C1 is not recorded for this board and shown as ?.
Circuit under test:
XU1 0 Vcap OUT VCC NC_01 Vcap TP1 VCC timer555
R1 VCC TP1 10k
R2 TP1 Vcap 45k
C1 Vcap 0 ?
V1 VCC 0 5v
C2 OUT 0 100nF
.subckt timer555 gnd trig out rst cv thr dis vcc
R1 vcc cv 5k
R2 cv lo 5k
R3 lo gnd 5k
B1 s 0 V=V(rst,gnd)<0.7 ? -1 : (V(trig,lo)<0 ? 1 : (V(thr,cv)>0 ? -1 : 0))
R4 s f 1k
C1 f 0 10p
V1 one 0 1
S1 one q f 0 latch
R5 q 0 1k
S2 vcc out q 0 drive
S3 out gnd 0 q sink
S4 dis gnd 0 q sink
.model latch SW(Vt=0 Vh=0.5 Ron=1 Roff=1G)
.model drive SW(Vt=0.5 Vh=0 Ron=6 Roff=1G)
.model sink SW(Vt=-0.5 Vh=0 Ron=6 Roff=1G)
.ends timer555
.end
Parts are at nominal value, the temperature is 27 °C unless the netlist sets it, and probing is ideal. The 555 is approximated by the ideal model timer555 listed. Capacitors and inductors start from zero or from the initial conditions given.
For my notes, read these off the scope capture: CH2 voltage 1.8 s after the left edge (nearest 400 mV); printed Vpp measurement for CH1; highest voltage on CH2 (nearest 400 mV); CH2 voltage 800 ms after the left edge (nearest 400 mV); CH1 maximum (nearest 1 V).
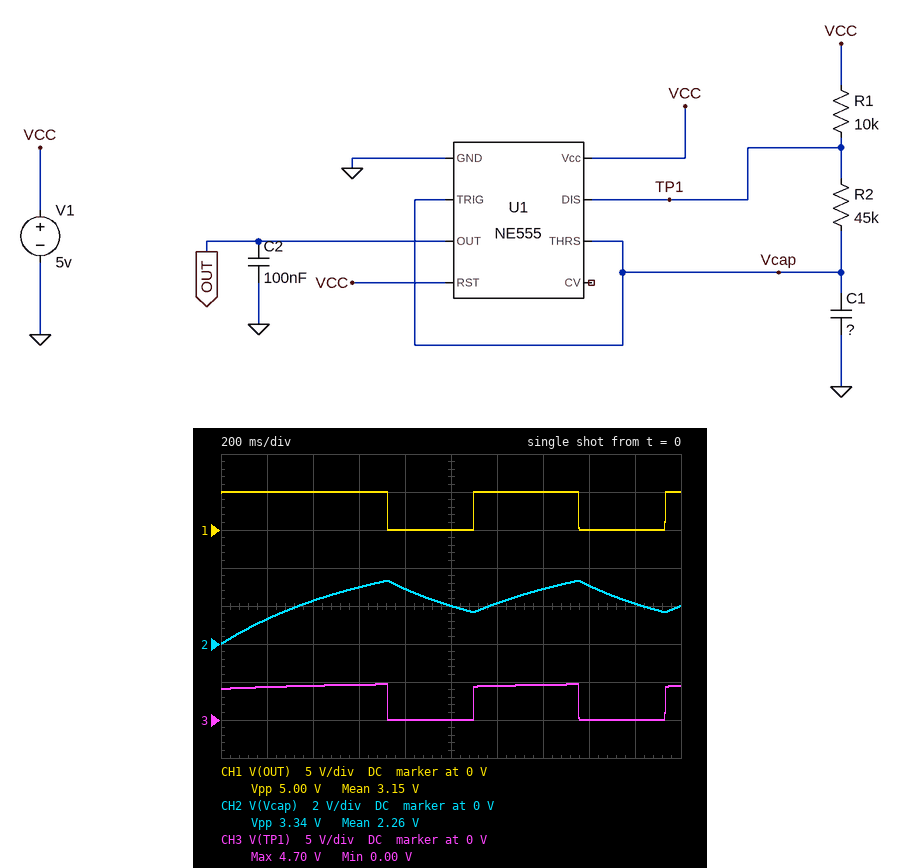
2.0 V
5.00 V
3.2 V
2.8 V
5 V
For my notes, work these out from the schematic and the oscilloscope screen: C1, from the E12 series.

12 µF
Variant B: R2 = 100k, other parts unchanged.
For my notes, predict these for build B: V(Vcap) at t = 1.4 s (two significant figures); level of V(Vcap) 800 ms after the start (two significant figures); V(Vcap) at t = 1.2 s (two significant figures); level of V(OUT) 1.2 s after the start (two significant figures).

3.3 V
2.3 V
3.0 V
5.0 V
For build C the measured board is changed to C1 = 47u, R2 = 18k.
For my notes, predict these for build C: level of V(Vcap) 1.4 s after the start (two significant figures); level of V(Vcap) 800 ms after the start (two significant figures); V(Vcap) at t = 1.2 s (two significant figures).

3.3 V
2.3 V
3.0 V
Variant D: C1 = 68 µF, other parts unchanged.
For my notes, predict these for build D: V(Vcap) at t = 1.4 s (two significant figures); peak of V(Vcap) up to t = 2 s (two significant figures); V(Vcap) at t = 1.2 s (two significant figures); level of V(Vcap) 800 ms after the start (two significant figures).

1.6 V
2.1 V
1.4 V
960 mV
